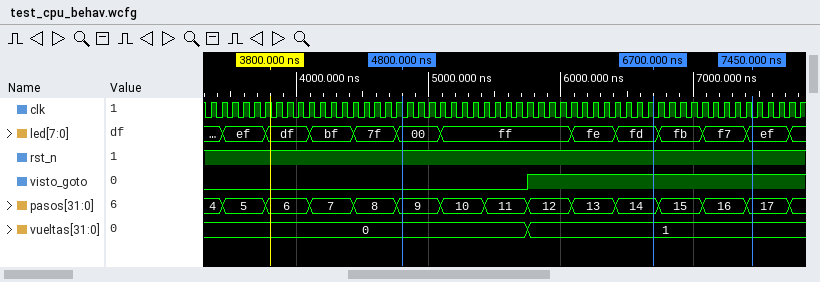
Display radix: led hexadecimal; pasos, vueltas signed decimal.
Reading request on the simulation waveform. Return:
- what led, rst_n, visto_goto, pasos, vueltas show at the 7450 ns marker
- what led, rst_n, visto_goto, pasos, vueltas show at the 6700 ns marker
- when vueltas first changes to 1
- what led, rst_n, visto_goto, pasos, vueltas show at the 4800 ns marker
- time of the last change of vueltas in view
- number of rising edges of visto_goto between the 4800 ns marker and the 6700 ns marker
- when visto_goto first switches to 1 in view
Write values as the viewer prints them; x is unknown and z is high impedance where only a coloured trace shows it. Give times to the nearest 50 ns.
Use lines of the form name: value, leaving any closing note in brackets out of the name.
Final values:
what led, rst_n, visto_goto, pasos, vueltas show at the 7450 ns marker: led=ef, rst_n=1, visto_goto=1, pasos=17, vueltas=1
what led, rst_n, visto_goto, pasos, vueltas show at the 6700 ns marker: led=fd, rst_n=1, visto_goto=1, pasos=14, vueltas=1
when vueltas first changes to 1: 5750 ns
what led, rst_n, visto_goto, pasos, vueltas show at the 4800 ns marker: led=00, rst_n=1, visto_goto=0, pasos=9, vueltas=0
time of the last change of vueltas in view: 5750 ns
number of rising edges of visto_goto between the 4800 ns marker and the 6700 ns marker: 1
when visto_goto first switches to 1 in view: 5750 ns
